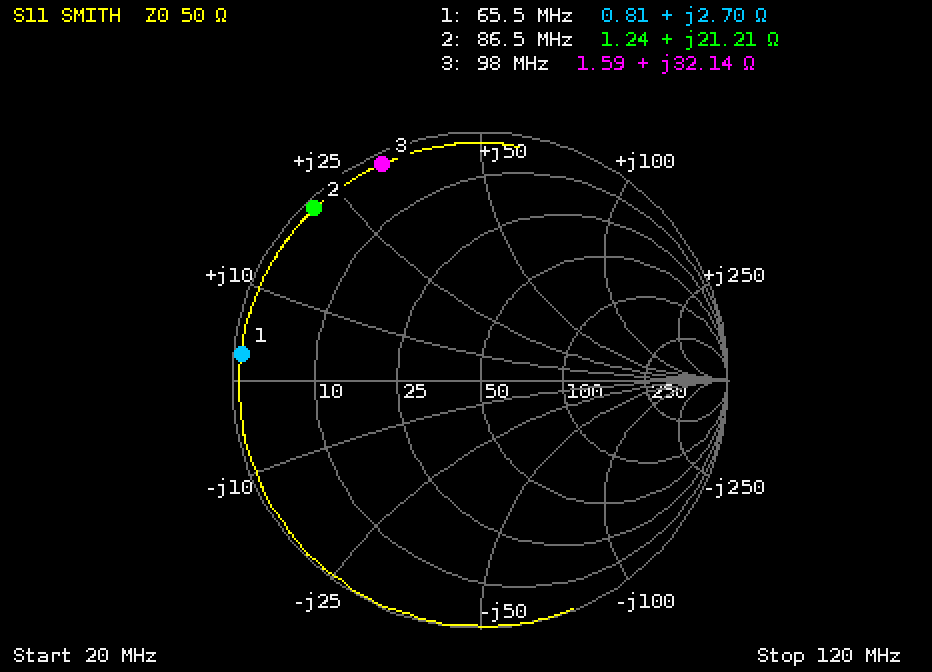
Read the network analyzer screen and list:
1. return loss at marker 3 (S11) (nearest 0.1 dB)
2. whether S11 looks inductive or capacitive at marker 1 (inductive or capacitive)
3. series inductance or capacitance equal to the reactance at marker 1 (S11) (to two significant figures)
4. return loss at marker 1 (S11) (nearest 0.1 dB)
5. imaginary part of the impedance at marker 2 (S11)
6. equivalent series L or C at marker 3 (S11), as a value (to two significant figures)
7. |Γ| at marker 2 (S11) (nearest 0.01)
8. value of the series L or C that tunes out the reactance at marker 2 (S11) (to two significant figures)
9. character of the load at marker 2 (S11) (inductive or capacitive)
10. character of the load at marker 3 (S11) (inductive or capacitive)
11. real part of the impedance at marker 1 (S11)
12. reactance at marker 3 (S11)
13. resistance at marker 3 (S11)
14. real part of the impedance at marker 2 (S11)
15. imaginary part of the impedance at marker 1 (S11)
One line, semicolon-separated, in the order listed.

0.4 dB; inductive; 6.6 nH; 0.3 dB; +21.21 Ω; 52 nH; 0.96; 87 pF; inductive; inductive; 0.81 Ω; +32.14 Ω; 1.59 Ω; 1.24 Ω; +2.70 Ω
